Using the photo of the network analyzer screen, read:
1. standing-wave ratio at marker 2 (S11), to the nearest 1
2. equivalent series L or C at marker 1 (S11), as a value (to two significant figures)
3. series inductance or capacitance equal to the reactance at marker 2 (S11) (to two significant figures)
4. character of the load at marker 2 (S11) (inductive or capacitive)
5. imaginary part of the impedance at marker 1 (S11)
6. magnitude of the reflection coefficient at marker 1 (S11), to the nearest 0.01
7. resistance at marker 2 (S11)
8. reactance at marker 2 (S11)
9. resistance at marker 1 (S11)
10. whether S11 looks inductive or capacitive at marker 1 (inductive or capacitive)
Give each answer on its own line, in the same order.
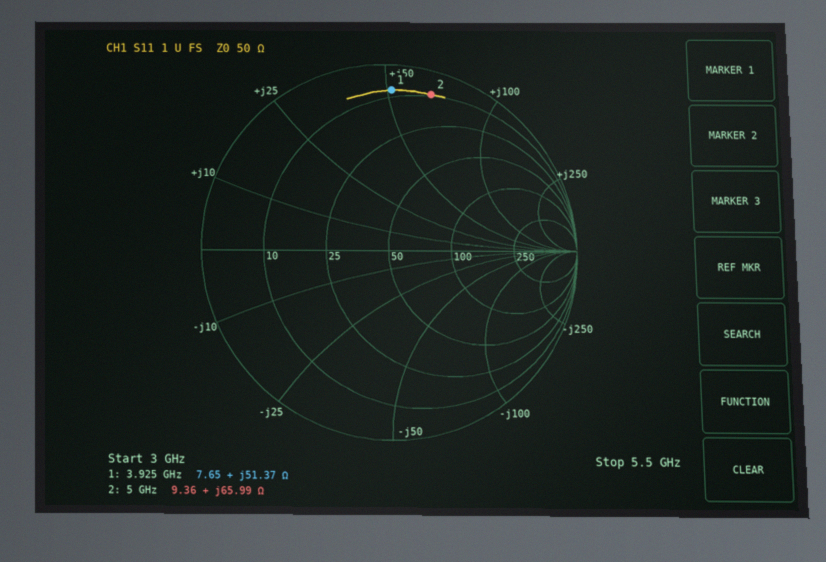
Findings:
15
2.1 nH
2.1 nH
inductive
+51.37 Ω
0.86
9.36 Ω
+65.99 Ω
7.65 Ω
inductive
